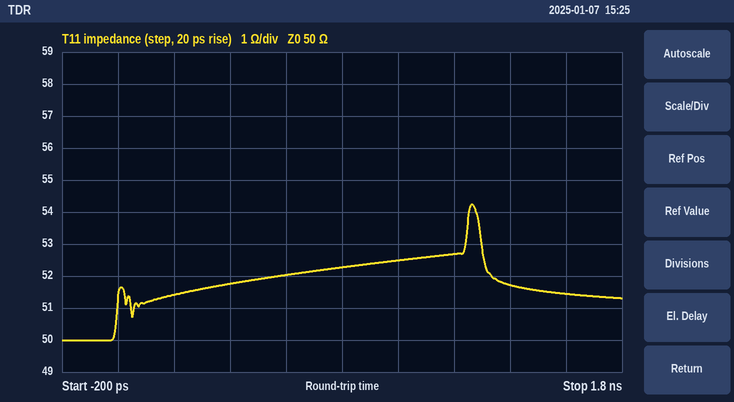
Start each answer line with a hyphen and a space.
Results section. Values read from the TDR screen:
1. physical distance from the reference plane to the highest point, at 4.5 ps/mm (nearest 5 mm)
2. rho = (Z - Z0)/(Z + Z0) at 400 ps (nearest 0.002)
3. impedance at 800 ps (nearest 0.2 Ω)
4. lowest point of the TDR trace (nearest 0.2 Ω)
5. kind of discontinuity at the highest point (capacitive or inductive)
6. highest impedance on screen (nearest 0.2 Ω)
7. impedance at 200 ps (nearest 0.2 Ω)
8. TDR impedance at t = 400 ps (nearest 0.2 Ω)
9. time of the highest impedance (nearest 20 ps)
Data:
- 140 mm
- +0.018
- 52.2 Ω
- 50.0 Ω
- inductive
- 54.2 Ω
- 51.4 Ω
- 51.8 Ω
- 1.26 ns
